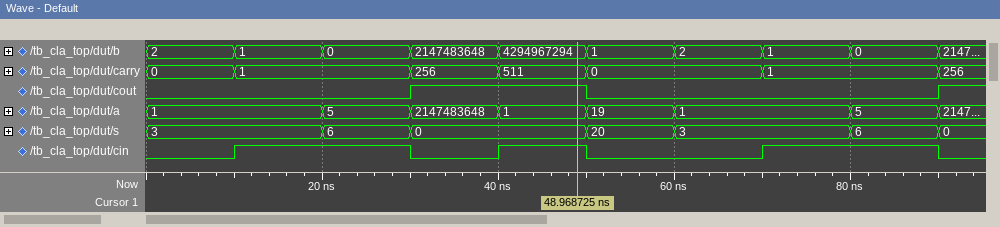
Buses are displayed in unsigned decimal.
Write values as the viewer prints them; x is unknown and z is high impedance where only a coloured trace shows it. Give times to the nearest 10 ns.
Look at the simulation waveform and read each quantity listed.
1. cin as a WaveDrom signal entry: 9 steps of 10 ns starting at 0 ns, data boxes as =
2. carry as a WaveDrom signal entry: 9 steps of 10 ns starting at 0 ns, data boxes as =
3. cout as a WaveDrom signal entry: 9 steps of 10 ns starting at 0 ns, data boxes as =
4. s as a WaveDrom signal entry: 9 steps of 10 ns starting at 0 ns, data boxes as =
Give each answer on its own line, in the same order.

{name: 'cin', wave: '01.010.1.'}
{name: 'carry', wave: '==.===.=.', data: '0 1 256 511 0 1'}
{name: 'cout', wave: '0..1.0...'}
{name: 's', wave: '=.==.==.=', data: '3 6 0 20 3 6'}
